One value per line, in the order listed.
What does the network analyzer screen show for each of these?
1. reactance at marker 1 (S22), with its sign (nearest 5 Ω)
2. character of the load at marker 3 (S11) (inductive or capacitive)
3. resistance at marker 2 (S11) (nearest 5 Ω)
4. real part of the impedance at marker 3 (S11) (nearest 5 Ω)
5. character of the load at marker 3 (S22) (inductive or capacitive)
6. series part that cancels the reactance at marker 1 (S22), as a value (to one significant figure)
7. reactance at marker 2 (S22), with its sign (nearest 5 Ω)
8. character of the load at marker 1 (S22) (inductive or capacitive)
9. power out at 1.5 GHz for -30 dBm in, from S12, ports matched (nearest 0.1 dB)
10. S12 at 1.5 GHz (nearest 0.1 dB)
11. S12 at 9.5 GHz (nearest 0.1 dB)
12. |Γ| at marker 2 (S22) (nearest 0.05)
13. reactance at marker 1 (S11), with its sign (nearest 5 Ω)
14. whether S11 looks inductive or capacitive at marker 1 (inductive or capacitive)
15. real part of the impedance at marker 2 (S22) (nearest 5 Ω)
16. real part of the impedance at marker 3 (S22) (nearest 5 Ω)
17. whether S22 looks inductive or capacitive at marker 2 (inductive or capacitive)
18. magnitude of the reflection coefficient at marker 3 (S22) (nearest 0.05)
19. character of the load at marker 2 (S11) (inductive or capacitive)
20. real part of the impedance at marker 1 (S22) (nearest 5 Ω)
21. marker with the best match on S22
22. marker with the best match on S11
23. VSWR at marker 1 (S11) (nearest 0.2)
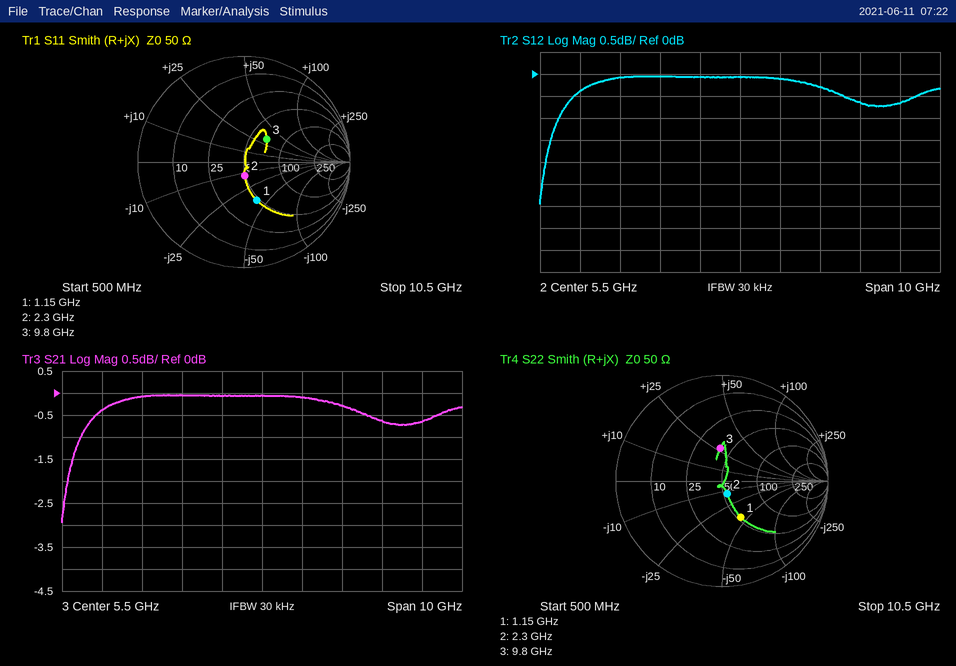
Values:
-45 Ω
inductive
50 Ω
70 Ω
inductive
6 nH
-15 Ω
capacitive
-30.4 dBm
-0.4 dB
-0.7 dB
0.15
-40 Ω
capacitive
55 Ω
40 Ω
capacitive
0.30
capacitive
55 Ω
marker 2
marker 2
2.2
